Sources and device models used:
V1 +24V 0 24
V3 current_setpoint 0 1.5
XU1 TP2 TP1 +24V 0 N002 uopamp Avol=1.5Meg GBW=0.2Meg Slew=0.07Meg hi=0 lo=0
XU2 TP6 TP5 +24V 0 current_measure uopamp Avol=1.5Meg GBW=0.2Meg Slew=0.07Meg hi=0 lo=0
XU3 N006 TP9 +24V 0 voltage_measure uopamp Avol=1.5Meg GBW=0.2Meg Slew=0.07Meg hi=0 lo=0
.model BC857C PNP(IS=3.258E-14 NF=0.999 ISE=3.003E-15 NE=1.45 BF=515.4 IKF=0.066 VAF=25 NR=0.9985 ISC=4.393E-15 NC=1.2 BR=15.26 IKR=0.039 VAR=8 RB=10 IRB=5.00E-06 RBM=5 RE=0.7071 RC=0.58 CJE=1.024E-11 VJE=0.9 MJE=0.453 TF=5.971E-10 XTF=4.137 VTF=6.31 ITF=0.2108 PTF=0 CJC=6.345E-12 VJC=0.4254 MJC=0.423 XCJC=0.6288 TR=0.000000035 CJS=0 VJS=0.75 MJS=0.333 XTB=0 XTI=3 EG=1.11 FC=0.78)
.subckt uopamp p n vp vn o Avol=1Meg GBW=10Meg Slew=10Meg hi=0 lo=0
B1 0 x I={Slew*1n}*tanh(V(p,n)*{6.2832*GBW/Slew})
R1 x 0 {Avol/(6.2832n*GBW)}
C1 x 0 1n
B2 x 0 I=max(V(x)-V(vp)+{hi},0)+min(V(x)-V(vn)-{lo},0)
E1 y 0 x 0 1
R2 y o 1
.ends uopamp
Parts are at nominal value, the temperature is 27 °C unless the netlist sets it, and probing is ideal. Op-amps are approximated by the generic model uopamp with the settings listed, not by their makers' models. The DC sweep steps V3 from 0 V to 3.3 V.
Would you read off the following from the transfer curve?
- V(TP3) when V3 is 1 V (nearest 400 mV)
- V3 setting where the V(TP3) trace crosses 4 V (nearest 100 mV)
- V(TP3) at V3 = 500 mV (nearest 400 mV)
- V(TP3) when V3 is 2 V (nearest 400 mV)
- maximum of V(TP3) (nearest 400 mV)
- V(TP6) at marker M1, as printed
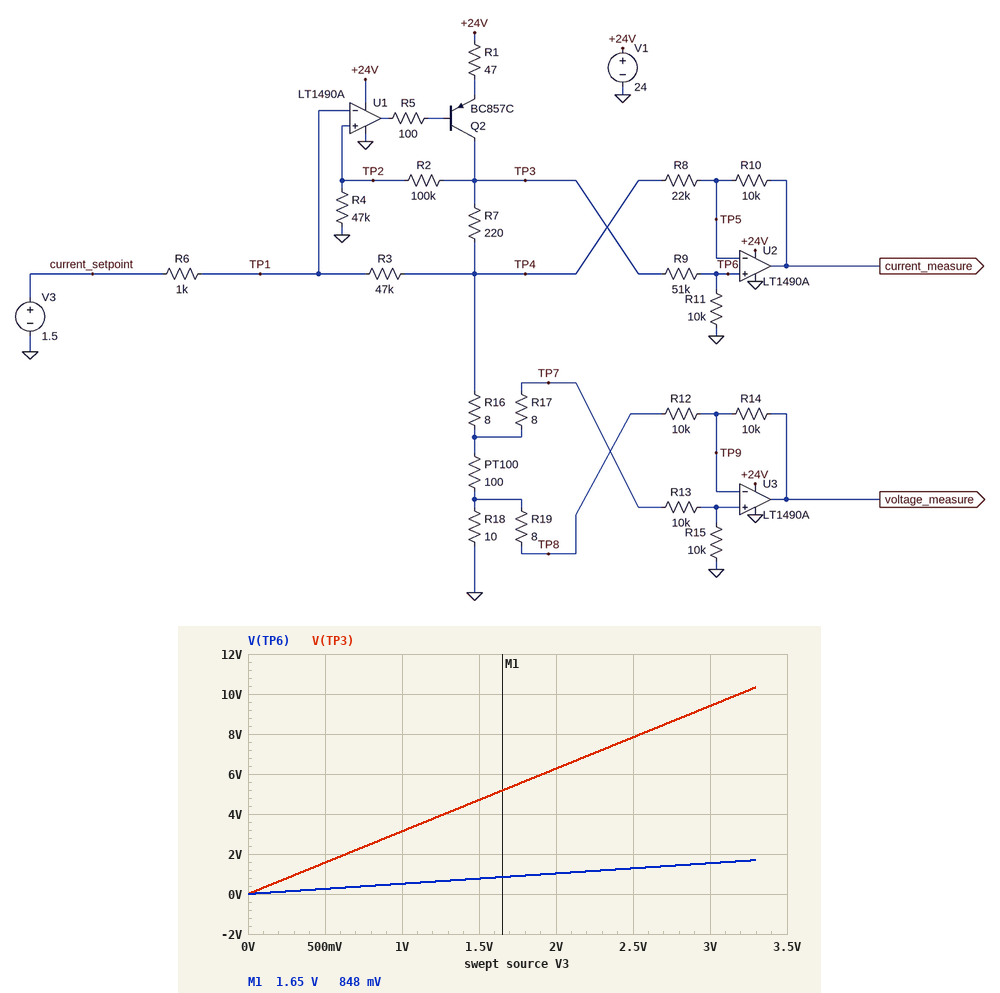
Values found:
3.2 V
1.3 V
1.6 V
6.4 V
10.4 V
848 mV
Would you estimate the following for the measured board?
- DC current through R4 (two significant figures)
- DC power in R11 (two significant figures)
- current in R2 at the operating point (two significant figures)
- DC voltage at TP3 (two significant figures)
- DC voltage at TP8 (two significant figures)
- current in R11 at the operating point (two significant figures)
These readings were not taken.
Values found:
32 µA
59 µW
32 µA
4.7 V
140 mV
77 µA
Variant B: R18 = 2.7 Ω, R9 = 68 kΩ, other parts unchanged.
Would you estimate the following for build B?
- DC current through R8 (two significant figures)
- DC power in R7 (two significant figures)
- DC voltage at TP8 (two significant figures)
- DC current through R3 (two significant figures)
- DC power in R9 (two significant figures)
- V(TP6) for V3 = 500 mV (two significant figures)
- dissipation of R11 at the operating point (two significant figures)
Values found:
44 µA
45 mW
39 mV
1.3 µA
250 µW
200 mV
36 µW
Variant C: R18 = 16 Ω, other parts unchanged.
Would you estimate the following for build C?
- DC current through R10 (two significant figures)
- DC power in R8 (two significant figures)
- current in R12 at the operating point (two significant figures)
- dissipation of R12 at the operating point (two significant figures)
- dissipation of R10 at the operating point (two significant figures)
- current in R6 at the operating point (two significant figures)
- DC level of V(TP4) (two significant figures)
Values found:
42 µA
38 µW
57 µA
32 µW
17 µW
3.9 µA
1.7 V
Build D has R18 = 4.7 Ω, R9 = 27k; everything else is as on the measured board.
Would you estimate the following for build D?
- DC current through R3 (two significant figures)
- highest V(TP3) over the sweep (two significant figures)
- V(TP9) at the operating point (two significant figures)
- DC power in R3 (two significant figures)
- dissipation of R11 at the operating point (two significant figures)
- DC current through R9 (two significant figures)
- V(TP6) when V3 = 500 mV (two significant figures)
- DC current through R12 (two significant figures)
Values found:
1.8 µA
10 V
740 mV
150 nW
160 µW
130 µA
420 mV
67 µA
